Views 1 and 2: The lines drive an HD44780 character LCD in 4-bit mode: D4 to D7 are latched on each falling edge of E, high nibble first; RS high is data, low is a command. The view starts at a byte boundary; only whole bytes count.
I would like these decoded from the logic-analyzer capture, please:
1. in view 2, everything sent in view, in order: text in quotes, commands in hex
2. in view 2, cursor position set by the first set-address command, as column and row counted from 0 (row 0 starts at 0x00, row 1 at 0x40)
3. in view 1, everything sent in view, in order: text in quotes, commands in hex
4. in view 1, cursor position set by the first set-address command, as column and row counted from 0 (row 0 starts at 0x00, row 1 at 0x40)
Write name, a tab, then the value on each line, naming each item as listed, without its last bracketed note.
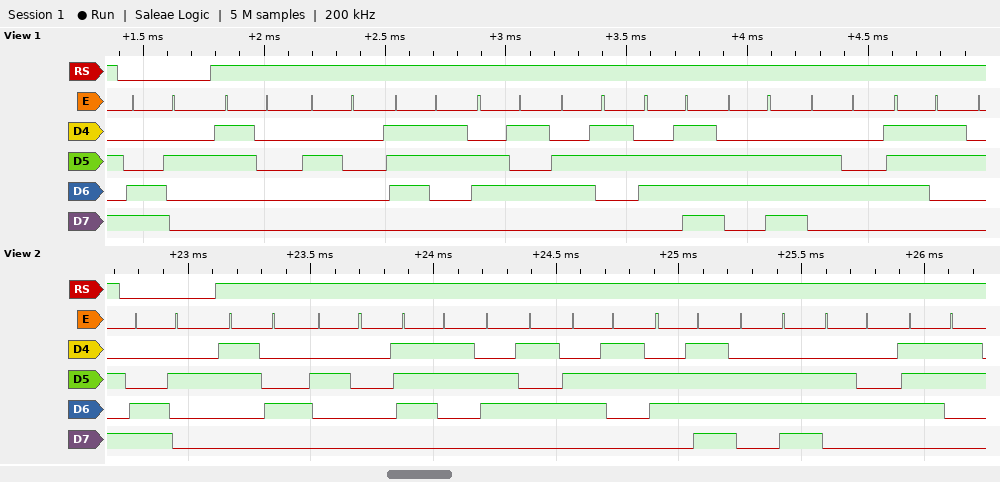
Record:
in view 2, everything sent in view, in order: text in quotes, commands in hex	0xC2 "4 seconds"
in view 2, cursor position set by the first set-address command, as column and row counted from 0	column 2, row 1
in view 1, everything sent in view, in order: text in quotes, commands in hex	0xC2 "0 seconds"
in view 1, cursor position set by the first set-address command, as column and row counted from 0	column 2, row 1
